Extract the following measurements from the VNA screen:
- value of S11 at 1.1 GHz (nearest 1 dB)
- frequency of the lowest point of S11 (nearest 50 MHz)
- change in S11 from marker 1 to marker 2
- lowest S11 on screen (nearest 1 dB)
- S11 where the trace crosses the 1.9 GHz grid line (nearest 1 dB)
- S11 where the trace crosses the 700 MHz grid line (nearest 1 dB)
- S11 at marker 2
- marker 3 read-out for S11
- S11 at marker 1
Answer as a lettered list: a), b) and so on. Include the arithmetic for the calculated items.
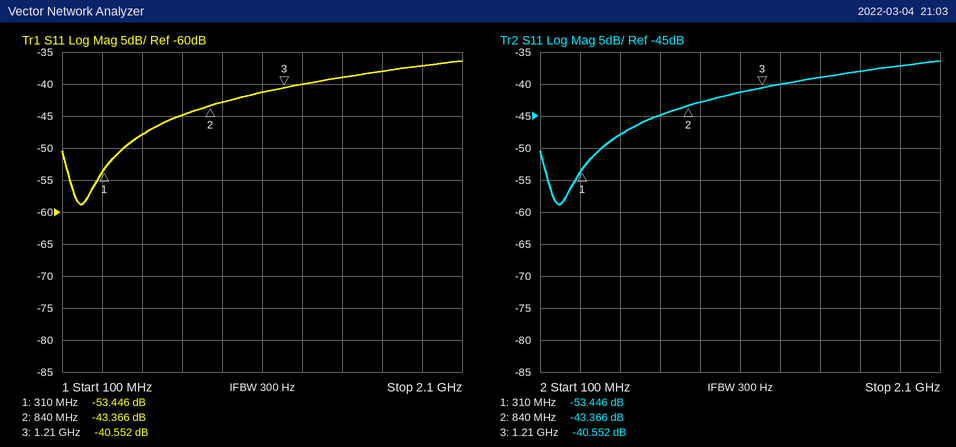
a) -41 dB
b) 200 MHz
c) -43.366 − (-53.446) = 10.080 dB
d) -59 dB
e) -37 dB
f) -45 dB
g) -43.366 dB
h) -40.552 dB
i) -53.446 dB
